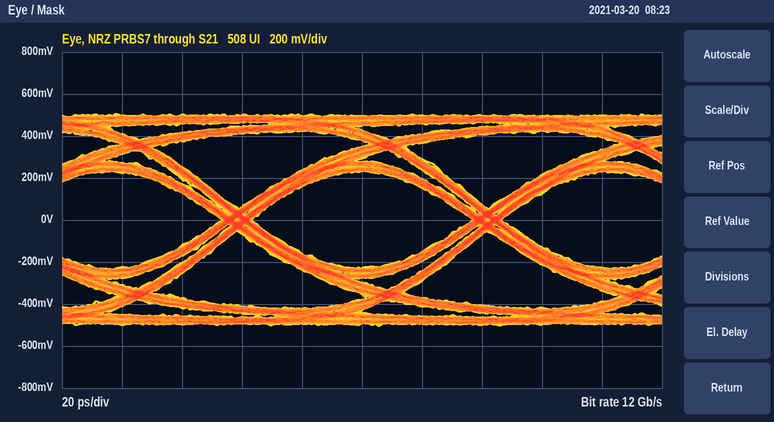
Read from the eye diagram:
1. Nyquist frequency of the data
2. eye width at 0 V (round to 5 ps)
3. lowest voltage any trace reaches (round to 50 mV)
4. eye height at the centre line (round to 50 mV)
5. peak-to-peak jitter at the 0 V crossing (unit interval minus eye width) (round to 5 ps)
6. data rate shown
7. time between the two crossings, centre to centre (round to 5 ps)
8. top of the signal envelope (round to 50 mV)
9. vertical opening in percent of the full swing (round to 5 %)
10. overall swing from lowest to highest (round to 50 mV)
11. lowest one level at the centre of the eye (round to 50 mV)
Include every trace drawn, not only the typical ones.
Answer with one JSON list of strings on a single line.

["6 GHz", "75 ps", "-500 mV", "450 mV", "10 ps", "12 Gb/s", "85 ps", "500 mV", "45 %", "1.00 V", "250 mV"]
